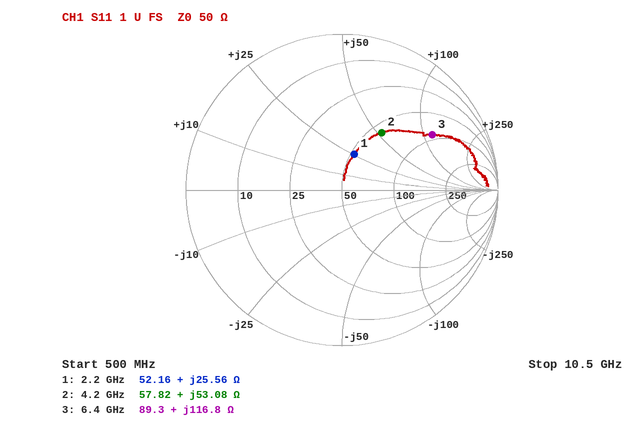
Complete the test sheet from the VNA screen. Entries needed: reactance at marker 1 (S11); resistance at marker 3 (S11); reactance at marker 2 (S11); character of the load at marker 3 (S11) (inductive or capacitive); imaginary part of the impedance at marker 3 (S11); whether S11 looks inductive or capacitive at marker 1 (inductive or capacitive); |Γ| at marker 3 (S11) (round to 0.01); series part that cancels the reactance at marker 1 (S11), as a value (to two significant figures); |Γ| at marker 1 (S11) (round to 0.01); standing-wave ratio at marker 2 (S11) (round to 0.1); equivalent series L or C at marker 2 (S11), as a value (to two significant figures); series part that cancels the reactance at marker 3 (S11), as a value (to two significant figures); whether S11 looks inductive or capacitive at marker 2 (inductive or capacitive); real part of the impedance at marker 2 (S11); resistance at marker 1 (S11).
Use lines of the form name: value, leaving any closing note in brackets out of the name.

reactance at marker 1: +25.56 Ω
resistance at marker 3: 89.3 Ω
reactance at marker 2: +53.08 Ω
character of the load at marker 3 (S11): inductive
imaginary part of the impedance at marker 3: +116.8 Ω
whether S11 looks inductive or capacitive at marker 1: inductive
|Γ| at marker 3 (S11): 0.68
series part that cancels the reactance at marker 1 (S11), as a value: 2.8 pF
|Γ| at marker 1 (S11): 0.24
standing-wave ratio at marker 2 (S11): 2.6
equivalent series L or C at marker 2 (S11), as a value: 2.0 nH
series part that cancels the reactance at marker 3 (S11), as a value: 210 fF
whether S11 looks inductive or capacitive at marker 2: inductive
real part of the impedance at marker 2: 57.82 Ω
resistance at marker 1: 52.16 Ω
